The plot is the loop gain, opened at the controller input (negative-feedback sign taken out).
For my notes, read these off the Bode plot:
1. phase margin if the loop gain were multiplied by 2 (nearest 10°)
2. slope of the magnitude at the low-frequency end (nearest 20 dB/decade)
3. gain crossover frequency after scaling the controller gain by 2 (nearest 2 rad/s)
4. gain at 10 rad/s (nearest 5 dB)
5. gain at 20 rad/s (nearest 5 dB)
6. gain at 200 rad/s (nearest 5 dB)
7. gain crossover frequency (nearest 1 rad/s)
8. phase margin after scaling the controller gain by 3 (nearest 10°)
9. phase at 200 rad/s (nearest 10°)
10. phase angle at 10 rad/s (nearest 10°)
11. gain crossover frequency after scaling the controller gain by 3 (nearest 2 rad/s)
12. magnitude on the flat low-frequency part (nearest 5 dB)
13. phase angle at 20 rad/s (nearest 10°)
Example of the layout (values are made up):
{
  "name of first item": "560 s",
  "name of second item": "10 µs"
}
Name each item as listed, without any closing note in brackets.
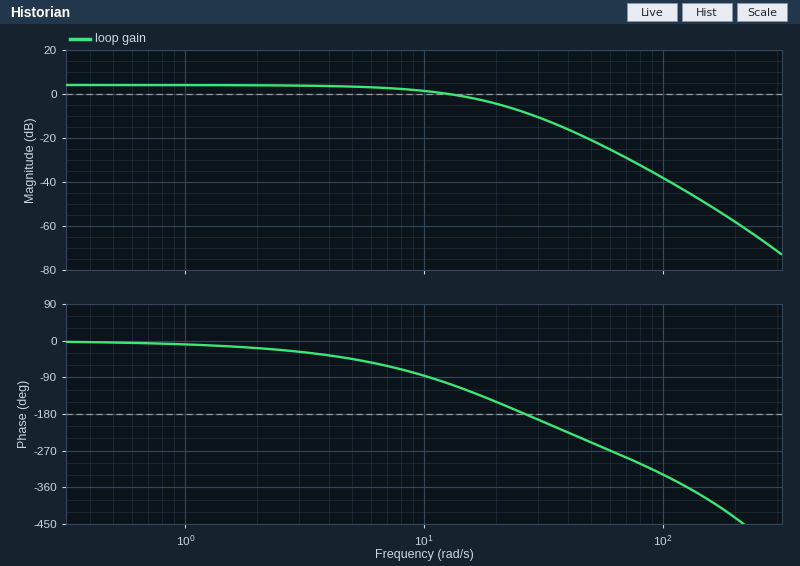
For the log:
{
  "phase margin if the loop gain were multiplied by 2": "20°",
  "slope of the magnitude at the low-frequency end": "0 dB/decade",
  "gain crossover frequency after scaling the controller gain by 2": "22 rad/s",
  "gain at 10 rad/s": "0 dB",
  "gain at 20 rad/s": "-5 dB",
  "gain at 200 rad/s": "-60 dB",
  "gain crossover frequency": "13 rad/s",
  "phase margin after scaling the controller gain by 3": "-10°",
  "phase at 200 rad/s": "-430°",
  "phase angle at 10 rad/s": "-90°",
  "gain crossover frequency after scaling the controller gain by 3": "28 rad/s",
  "magnitude on the flat low-frequency part": "5 dB",
  "phase angle at 20 rad/s": "-150°"
}
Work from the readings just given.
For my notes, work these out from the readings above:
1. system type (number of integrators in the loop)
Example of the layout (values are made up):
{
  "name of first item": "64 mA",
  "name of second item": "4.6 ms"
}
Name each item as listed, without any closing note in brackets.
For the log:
{
  "system type": "0"
}
